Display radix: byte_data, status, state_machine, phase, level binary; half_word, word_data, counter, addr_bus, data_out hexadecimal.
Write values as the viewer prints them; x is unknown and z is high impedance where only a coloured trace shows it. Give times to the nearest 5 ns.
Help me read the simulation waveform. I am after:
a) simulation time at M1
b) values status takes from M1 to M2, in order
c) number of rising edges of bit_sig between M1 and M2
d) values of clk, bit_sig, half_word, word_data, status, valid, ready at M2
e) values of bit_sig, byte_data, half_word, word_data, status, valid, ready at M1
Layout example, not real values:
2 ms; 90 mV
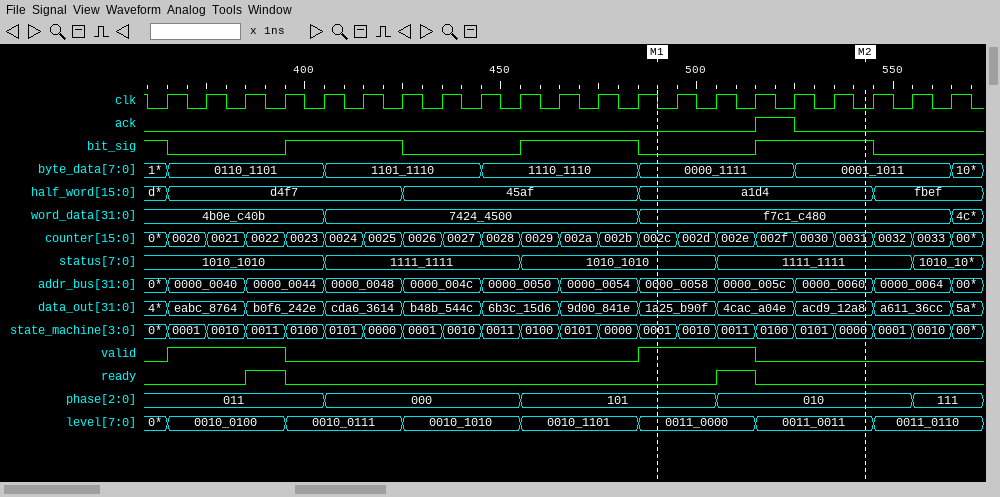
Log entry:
490 ns; 1010_1010, 1111_1111; 1; clk=0, bit_sig=1, half_word=a1d4, word_data=f7c1_c480, status=1111_1111, valid=0, ready=0; bit_sig=0, byte_data=0000_1111, half_word=a1d4, word_data=f7c1_c480, status=1010_1010, valid=1, ready=0
